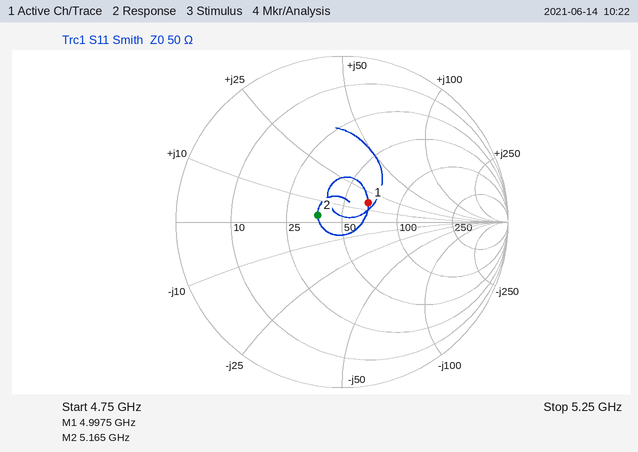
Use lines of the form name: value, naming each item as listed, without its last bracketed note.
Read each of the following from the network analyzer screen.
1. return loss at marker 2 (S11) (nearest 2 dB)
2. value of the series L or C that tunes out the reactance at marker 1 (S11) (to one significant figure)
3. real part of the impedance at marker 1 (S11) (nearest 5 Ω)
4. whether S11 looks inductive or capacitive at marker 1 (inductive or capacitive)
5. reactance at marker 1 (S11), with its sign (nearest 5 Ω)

return loss at marker 2 (S11): 16 dB
value of the series L or C that tunes out the reactance at marker 1 (S11): 2 pF
real part of the impedance at marker 1 (S11): 65 Ω
whether S11 looks inductive or capacitive at marker 1: inductive
reactance at marker 1 (S11), with its sign: +15 Ω
